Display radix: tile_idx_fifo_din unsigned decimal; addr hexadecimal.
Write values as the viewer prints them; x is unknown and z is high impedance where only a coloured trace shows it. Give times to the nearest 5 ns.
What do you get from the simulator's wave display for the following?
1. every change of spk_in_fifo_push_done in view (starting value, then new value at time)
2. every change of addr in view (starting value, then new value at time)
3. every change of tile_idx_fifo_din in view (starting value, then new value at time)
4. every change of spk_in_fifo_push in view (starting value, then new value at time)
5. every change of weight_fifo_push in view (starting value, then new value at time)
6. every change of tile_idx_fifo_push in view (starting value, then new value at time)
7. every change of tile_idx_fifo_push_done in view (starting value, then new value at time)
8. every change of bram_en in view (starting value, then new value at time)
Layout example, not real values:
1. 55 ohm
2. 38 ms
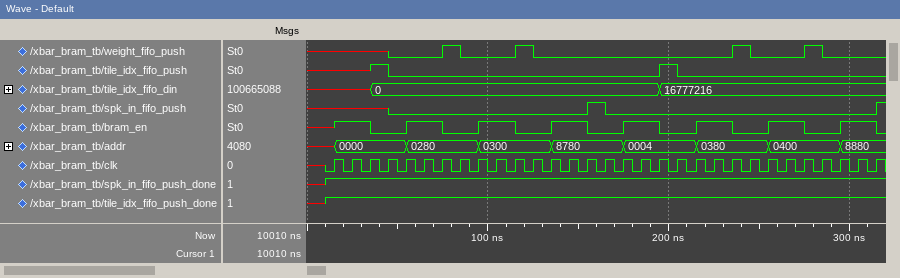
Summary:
1. x, 1 at 10 ns
2. x, 0000 at 15 ns, 0280 at 55 ns, 0300 at 95 ns, 8780 at 135 ns, 0004 at 175 ns, 0380 at 215 ns, 0400 at 255 ns, 8880 at 295 ns
3. x, 0 at 35 ns, 16777216 at 195 ns
4. x, 0 at 45 ns, 1 at 155 ns, 0 at 165 ns, 1 at 315 ns
5. x, 0 at 45 ns, 1 at 75 ns, 0 at 85 ns, 1 at 115 ns, 0 at 125 ns, 1 at 235 ns, 0 at 245 ns, 1 at 275 ns, 0 at 285 ns
6. x, 1 at 35 ns, 0 at 45 ns, 1 at 195 ns, 0 at 205 ns
7. x, 1 at 10 ns
8. x, 1 at 15 ns, 0 at 35 ns, 1 at 55 ns, 0 at 75 ns, 1 at 95 ns, 0 at 115 ns, 1 at 135 ns, 0 at 155 ns, 1 at 175 ns, 0 at 195 ns, 1 at 215 ns, 0 at 235 ns, 1 at 255 ns, 0 at 275 ns, 1 at 295 ns, 0 at 315 ns
